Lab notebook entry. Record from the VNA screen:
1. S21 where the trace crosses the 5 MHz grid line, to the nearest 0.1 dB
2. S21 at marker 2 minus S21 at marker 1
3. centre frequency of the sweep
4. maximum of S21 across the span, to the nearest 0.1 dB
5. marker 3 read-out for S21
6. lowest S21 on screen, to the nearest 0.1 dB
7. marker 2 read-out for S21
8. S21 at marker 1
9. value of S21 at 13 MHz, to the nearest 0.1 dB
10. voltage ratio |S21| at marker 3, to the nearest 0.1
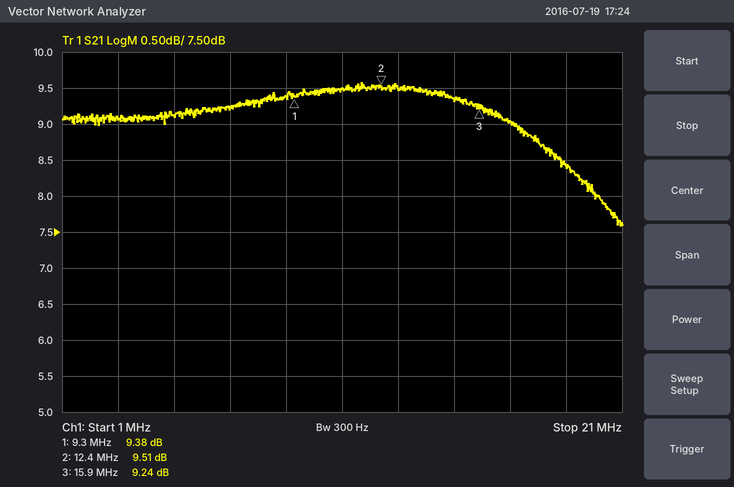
9.1 dB
0.13 dB
11 MHz
9.6 dB
9.24 dB
7.6 dB
9.51 dB
9.38 dB
9.5 dB
2.9
